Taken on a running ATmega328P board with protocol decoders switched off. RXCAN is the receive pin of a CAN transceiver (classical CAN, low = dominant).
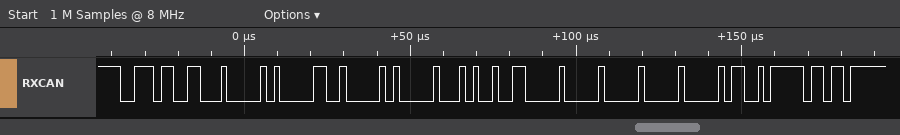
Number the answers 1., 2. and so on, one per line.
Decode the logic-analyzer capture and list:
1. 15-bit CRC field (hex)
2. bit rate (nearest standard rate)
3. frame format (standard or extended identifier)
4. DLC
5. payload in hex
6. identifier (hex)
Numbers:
1. 0x65FD
2. 500 kbit/s
3. standard
4. 8
5. 10 48 10 0A 4C 00 00 00
6. 0x3B3
